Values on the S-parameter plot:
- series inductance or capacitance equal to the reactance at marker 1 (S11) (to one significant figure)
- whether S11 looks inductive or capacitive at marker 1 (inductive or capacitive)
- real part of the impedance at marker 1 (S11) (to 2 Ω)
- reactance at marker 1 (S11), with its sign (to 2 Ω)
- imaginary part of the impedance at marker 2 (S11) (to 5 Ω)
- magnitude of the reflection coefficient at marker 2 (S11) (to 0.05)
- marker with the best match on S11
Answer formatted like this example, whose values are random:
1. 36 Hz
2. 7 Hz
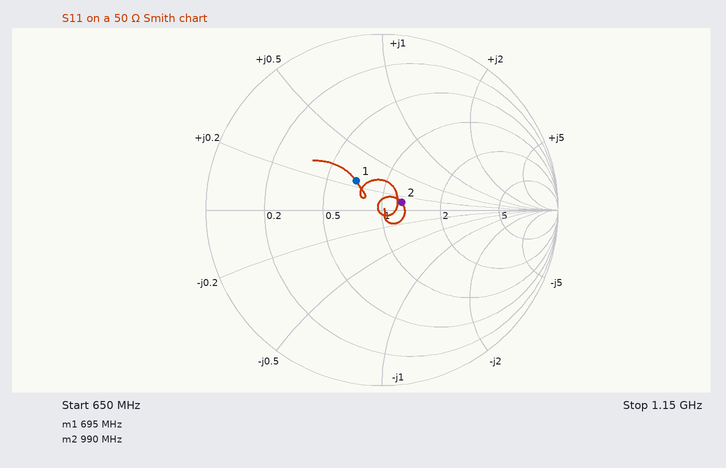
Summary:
1. 3 nH
2. inductive
3. 36 Ω
4. +12 Ω
5. +5 Ω
6. 0.10
7. marker 2
